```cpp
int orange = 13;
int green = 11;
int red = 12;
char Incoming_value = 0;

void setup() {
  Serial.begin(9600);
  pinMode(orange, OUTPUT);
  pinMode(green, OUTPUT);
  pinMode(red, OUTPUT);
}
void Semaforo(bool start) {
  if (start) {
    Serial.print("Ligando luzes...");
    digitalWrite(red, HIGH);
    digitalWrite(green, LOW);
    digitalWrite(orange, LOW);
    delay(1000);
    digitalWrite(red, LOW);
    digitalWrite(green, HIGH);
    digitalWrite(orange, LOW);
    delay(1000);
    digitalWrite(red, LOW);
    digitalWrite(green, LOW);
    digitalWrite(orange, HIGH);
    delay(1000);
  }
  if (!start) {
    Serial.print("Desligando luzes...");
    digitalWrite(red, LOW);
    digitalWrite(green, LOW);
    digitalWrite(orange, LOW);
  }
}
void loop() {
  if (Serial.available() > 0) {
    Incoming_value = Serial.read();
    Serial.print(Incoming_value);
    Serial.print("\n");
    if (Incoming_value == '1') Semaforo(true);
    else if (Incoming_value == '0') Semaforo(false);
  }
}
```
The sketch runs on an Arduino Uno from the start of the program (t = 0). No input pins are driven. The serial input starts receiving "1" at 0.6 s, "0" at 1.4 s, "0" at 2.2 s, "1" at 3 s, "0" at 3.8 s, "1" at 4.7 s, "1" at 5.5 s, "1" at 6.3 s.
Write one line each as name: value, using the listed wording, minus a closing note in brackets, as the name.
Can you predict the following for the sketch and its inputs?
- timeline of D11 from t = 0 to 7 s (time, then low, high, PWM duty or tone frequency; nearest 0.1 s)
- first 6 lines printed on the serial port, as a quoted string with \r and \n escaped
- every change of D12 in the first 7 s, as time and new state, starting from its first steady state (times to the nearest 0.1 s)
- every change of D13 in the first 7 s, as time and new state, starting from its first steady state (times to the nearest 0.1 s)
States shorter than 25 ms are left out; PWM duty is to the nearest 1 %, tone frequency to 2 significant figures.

timeline of D11 from t = 0 to 7 s: 0 s low; 1.6 s high; 2.6 s low; 4.6 s high; 5.6 s low
first 6 lines printed on the serial port, as a quoted string with \r and \n escaped: "1\nLigando luzes...0\nDesligando luzes...0\nDesligando luzes...1\nLigando luzes...0\nDesligando luzes...1\n"
every change of D12 in the first 7 s, as time and new state, starting from its first steady state: 0 s low; 0.6 s high; 1.6 s low; 3.6 s high; 4.6 s low; 6.6 s high
every change of D13 in the first 7 s, as time and new state, starting from its first steady state: 0 s low; 2.6 s high; 3.6 s low; 5.6 s high; 6.6 s low
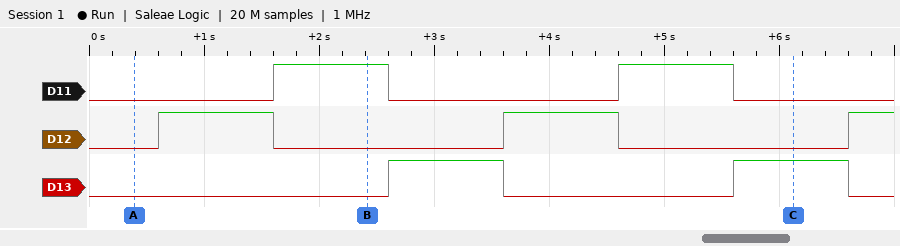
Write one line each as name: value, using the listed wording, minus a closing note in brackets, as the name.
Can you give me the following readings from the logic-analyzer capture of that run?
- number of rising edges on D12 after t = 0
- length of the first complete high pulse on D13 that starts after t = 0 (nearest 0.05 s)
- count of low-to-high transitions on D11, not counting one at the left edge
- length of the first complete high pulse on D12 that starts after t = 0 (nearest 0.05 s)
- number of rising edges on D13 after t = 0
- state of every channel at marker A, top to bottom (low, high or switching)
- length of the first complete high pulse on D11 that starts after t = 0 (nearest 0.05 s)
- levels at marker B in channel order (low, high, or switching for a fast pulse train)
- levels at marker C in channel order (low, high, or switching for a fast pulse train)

number of rising edges on D12 after t = 0: 3
length of the first complete high pulse on D13 that starts after t = 0: 1.00 s
count of low-to-high transitions on D11, not counting one at the left edge: 2
length of the first complete high pulse on D12 that starts after t = 0: 1.00 s
number of rising edges on D13 after t = 0: 2
state of every channel at marker A, top to bottom: D11 low, D12 low, D13 low
length of the first complete high pulse on D11 that starts after t = 0: 1.00 s
levels at marker B in channel order: D11 high, D12 low, D13 low
levels at marker C in channel order: D11 low, D12 low, D13 high
